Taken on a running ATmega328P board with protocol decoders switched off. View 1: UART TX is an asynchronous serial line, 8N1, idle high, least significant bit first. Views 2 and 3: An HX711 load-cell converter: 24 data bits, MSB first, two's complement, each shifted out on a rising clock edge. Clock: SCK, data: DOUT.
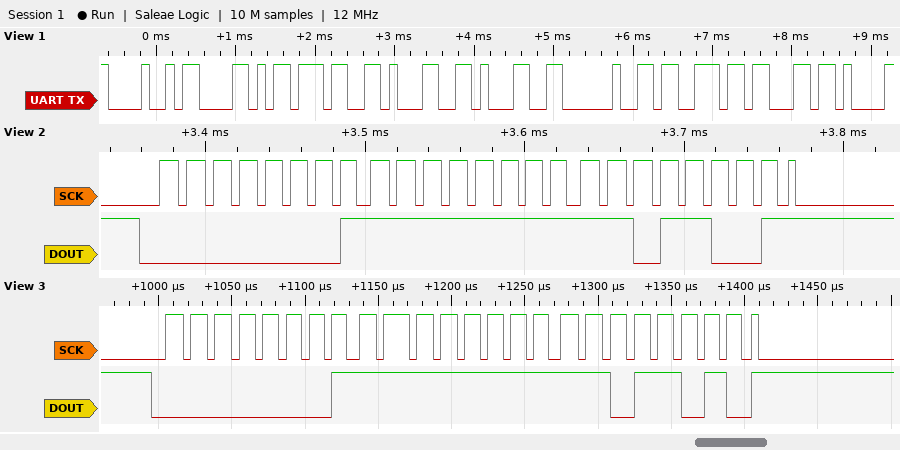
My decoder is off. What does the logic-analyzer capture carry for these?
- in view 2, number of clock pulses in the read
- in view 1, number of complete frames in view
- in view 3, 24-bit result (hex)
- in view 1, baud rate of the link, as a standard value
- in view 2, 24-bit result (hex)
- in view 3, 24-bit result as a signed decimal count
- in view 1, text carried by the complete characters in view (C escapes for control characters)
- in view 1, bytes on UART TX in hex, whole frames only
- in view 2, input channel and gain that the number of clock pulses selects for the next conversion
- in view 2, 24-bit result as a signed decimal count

25
8
0x01FFDA
9600 baud
0x01FFD9
131034
"HX711 sc"
48 58 37 31 31 20 73 63
channel A, gain 128
131033
